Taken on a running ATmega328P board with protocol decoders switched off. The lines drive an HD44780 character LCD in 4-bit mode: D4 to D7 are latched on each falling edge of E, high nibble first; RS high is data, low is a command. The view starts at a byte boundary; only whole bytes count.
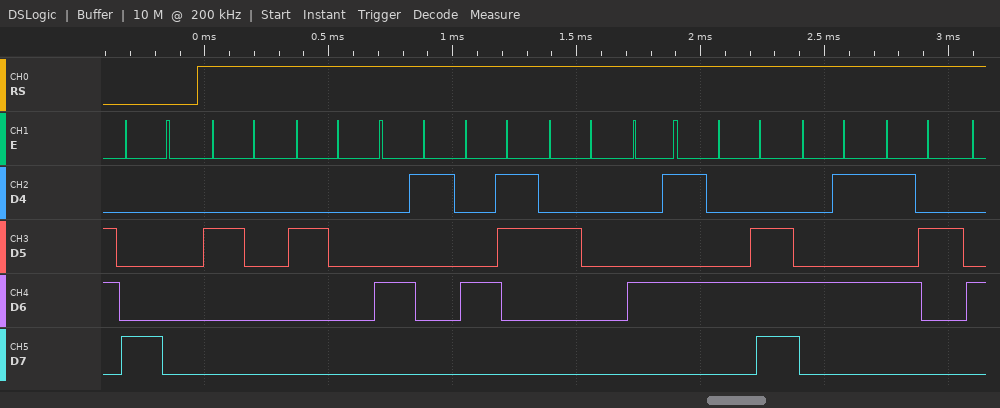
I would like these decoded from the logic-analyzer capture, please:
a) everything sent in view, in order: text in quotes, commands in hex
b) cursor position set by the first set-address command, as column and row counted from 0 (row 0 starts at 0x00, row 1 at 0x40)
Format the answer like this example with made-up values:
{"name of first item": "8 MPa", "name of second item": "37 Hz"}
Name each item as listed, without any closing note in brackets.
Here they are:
{"everything sent in view, in order: text in quotes, commands in hex": "0x80 \"  AC ENER\"", "cursor position set by the first set-address command, as column and row counted from 0": "column 0, row 0"}
